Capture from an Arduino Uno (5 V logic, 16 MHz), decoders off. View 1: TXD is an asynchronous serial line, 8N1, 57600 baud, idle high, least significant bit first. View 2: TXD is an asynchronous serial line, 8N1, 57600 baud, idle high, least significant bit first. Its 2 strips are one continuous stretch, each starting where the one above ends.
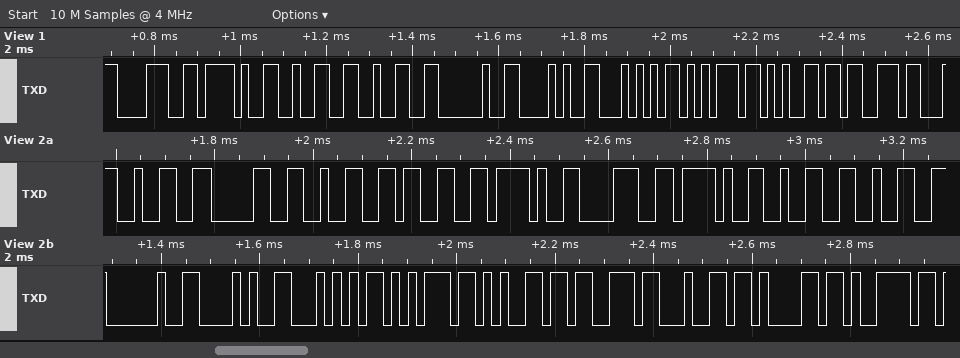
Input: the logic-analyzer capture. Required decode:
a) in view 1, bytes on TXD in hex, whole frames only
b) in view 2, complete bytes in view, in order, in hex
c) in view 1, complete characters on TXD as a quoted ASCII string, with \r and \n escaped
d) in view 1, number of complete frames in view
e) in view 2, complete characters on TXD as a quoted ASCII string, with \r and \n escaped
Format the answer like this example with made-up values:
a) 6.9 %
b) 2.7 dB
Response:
a) 38 2F 32 32 20 28 54 75 65 73
b) 32 30 32 33 2F 38 2F 32 32 20 28 54 75 65 73 64 61 79
c) "8/22 (Tues"
d) 10
e) "2023/8/22 (Tuesday"
